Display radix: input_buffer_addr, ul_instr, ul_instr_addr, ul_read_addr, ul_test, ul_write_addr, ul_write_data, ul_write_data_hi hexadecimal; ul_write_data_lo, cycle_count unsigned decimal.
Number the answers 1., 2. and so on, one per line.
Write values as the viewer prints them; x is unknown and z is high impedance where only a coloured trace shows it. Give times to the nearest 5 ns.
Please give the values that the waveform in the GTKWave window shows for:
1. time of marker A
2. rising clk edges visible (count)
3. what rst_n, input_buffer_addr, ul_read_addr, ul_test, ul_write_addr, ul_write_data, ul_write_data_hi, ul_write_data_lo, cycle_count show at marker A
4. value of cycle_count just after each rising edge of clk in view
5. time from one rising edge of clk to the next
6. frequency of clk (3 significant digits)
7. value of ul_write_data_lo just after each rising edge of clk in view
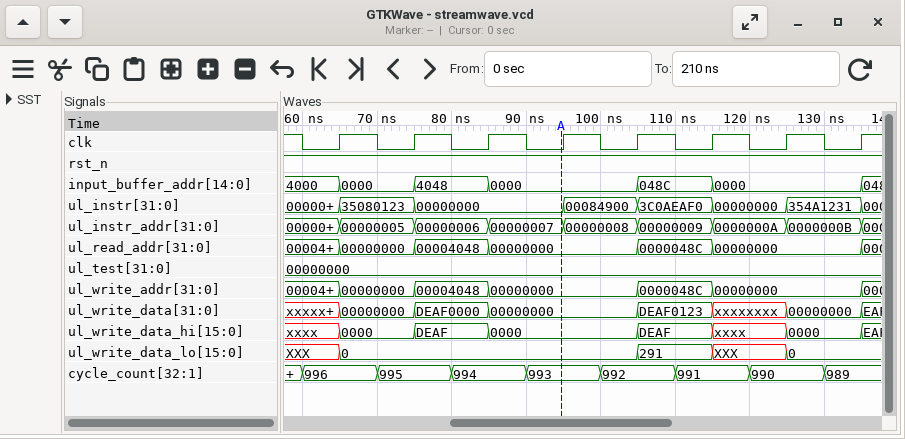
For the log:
1. 95 ns
2. 8
3. rst_n=1, input_buffer_addr=0000, ul_read_addr=00000000, ul_test=00000000, ul_write_addr=00000000, ul_write_data=00000000, ul_write_data_hi=0000, ul_write_data_lo=0, cycle_count=993
4. 996, 995, 994, 993, 992, 991, 990, 989
5. 10 ns
6. 100 MHz
7. 0, 0, 0, 0, 291, XXX, 0, 0
